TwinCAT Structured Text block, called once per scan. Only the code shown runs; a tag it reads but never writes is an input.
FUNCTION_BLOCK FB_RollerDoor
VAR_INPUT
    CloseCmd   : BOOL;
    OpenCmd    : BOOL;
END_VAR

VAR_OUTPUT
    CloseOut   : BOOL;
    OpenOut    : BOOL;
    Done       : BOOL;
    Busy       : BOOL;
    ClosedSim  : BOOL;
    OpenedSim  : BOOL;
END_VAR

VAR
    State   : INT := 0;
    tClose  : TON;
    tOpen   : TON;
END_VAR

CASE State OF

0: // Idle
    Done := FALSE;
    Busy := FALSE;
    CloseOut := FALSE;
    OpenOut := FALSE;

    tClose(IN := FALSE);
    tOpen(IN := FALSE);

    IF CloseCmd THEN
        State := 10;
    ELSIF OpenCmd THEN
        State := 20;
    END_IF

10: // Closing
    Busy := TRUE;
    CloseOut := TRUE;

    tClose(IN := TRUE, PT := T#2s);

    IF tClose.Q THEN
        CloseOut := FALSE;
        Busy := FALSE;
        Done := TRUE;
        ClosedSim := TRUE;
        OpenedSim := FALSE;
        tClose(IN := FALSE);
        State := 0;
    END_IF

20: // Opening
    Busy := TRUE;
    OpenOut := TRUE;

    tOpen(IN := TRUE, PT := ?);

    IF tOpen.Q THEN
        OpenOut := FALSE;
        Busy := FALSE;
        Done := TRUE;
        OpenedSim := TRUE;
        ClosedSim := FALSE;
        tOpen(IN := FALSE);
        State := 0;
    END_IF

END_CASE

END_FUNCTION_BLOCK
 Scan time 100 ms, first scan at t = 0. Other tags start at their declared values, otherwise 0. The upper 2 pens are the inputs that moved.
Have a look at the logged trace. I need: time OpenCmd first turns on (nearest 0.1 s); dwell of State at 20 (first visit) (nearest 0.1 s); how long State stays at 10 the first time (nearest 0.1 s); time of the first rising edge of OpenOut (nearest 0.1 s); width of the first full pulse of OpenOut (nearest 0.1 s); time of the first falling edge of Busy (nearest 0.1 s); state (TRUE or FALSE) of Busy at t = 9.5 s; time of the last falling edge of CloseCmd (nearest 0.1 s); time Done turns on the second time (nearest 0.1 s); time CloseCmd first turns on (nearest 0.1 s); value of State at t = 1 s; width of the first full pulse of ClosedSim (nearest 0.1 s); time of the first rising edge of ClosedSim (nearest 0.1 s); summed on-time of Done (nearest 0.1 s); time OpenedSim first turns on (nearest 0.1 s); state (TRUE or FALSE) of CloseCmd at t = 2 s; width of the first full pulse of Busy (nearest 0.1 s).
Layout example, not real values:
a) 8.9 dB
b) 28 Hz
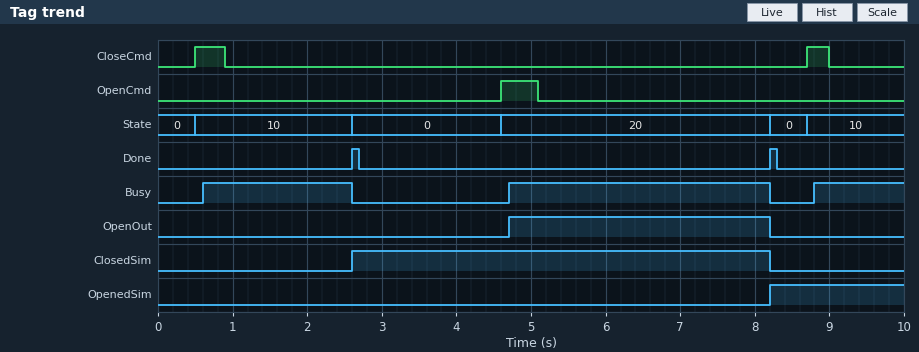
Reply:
a) 4.6 s
b) 3.6 s
c) 2.1 s
d) 4.7 s
e) 3.5 s
f) 2.6 s
g) TRUE
h) 9.0 s
i) 8.2 s
j) 0.5 s
k) 10
l) 5.6 s
m) 2.6 s
n) 0.2 s
o) 8.2 s
p) FALSE
q) 2.0 s
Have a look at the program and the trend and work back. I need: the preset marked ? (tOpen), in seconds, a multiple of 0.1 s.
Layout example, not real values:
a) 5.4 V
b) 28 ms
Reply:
a) 3.5 s
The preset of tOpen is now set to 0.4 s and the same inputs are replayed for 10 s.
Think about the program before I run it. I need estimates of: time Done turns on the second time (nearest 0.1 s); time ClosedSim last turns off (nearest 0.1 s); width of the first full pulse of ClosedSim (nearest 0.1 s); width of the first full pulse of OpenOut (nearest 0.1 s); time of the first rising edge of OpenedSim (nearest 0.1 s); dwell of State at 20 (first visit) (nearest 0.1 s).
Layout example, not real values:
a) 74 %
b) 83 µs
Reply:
a) 5.1 s
b) 5.1 s
c) 2.5 s
d) 0.4 s
e) 5.1 s
f) 0.5 s
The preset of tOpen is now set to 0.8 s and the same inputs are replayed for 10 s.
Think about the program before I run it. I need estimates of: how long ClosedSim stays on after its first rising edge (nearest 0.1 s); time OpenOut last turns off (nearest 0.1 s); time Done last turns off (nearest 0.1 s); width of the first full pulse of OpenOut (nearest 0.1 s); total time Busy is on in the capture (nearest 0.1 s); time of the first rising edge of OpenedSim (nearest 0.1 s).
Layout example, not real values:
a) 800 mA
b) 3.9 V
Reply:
a) 2.9 s
b) 5.5 s
c) 5.6 s
d) 0.8 s
e) 4.0 s
f) 5.5 s
